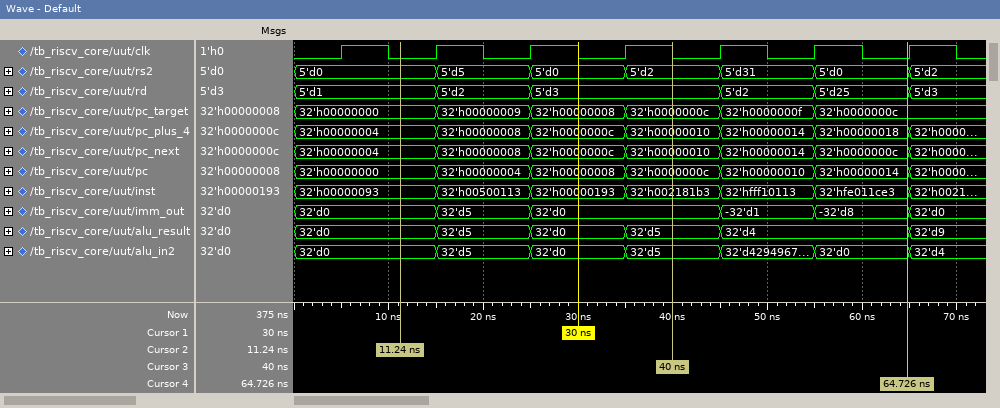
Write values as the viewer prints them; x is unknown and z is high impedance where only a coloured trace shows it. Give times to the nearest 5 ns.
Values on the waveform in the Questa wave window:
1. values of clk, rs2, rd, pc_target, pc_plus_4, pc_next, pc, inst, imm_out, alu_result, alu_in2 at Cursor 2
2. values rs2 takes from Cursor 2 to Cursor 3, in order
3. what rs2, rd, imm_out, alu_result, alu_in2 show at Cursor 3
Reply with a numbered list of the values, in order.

1. clk=0, rs2=5'd0, rd=5'd1, pc_target=32'h00000000, pc_plus_4=32'h00000004, pc_next=32'h00000004, pc=32'h00000000, inst=32'h00000093, imm_out=32'd0, alu_result=32'd0, alu_in2=32'd0
2. 5'd0, 5'd5, 5'd0, 5'd2
3. rs2=5'd2, rd=5'd3, imm_out=32'd0, alu_result=32'd5, alu_in2=32'd5
